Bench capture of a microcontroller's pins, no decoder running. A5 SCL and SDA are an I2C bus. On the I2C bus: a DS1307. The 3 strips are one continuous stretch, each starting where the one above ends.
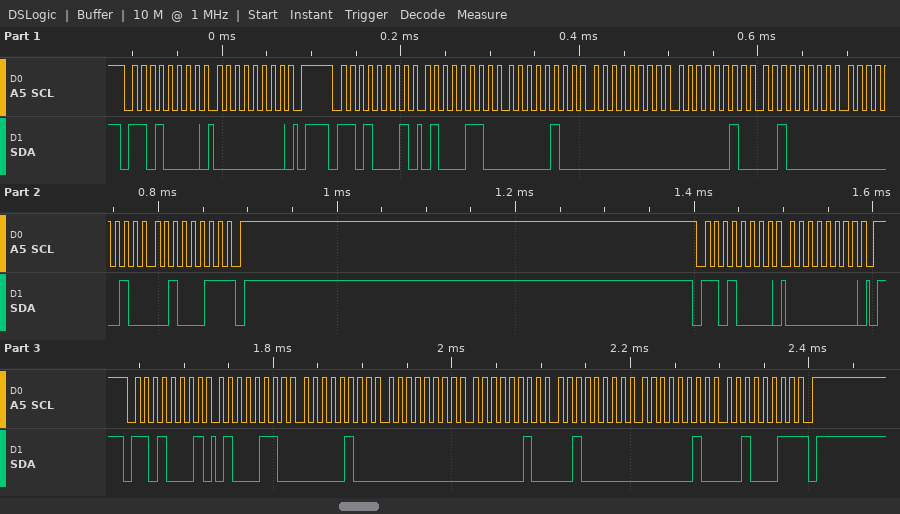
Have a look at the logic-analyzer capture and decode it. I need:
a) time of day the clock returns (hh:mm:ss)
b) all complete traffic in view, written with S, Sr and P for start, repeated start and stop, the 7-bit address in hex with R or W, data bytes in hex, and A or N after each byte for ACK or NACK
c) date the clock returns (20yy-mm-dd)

00:04:46
S 68W A 00 A P S 68R A 46 A 04 A 00 A 02 A 20 A 02 A 23 N P S 68W A 00 A P S 68R A 46 A 04 A 00 A 02 A 20 A 02 A 23 N P
2023-02-20
